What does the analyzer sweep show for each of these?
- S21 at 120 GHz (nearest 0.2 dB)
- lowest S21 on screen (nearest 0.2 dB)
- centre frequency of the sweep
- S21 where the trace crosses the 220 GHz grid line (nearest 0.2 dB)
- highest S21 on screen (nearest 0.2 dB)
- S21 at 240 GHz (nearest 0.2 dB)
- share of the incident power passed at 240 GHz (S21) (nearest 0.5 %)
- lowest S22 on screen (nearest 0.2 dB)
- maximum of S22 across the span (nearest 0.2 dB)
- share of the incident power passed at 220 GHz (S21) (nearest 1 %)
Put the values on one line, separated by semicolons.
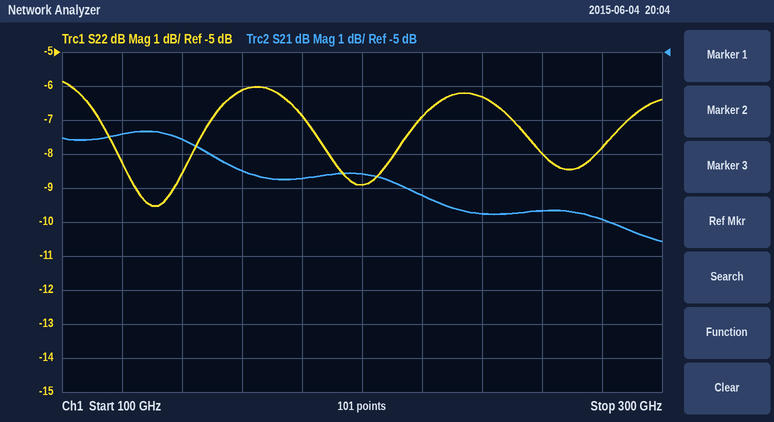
-7.4 dB; -10.6 dB; 200 GHz; -9.2 dB; -7.4 dB; -9.8 dB; 10.5 %; -9.6 dB; -5.8 dB; 12 %
